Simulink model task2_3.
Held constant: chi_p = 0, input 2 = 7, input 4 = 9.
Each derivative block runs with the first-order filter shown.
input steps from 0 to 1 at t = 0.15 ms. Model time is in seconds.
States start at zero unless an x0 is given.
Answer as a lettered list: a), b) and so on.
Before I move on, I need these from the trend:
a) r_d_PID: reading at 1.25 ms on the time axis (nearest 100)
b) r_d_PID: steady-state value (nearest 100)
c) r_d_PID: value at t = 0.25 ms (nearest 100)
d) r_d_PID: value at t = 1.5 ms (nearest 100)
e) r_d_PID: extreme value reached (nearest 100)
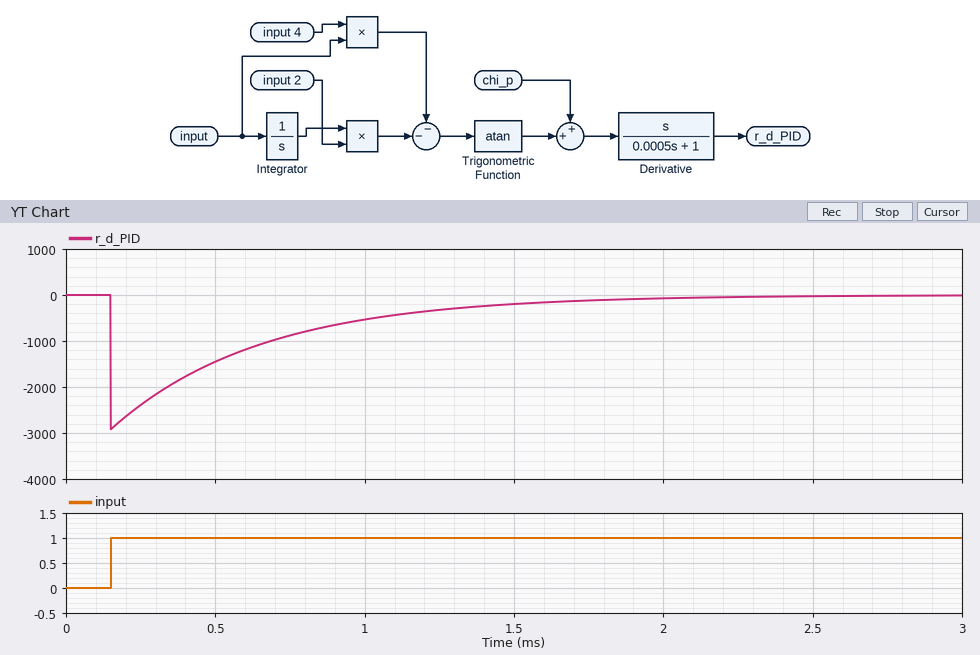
a) -300
b) 0
c) -2400
d) -200
e) -2900
